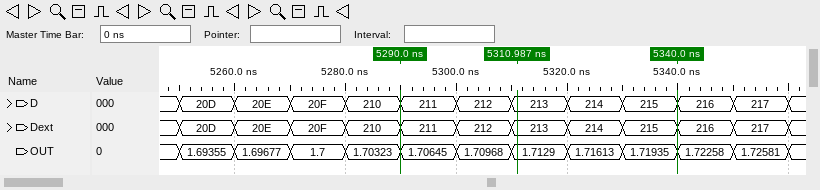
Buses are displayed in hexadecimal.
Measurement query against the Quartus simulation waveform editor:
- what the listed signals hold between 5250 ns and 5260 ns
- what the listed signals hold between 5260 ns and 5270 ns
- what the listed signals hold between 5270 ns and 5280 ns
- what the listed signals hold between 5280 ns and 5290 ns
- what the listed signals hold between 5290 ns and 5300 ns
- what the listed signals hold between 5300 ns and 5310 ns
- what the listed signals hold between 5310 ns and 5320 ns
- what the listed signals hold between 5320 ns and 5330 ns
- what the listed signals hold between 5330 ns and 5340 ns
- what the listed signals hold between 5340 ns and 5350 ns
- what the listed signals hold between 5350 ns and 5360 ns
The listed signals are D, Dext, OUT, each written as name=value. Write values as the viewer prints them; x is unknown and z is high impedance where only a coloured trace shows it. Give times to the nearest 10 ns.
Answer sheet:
D=20D, Dext=20D, OUT=1.69355
D=20E, Dext=20E, OUT=1.69677
D=20F, Dext=20F, OUT=1.7
D=210, Dext=210, OUT=1.70323
D=211, Dext=211, OUT=1.70645
D=212, Dext=212, OUT=1.70968
D=213, Dext=213, OUT=1.7129
D=214, Dext=214, OUT=1.71613
D=215, Dext=215, OUT=1.71935
D=216, Dext=216, OUT=1.72258
D=217, Dext=217, OUT=1.72581
